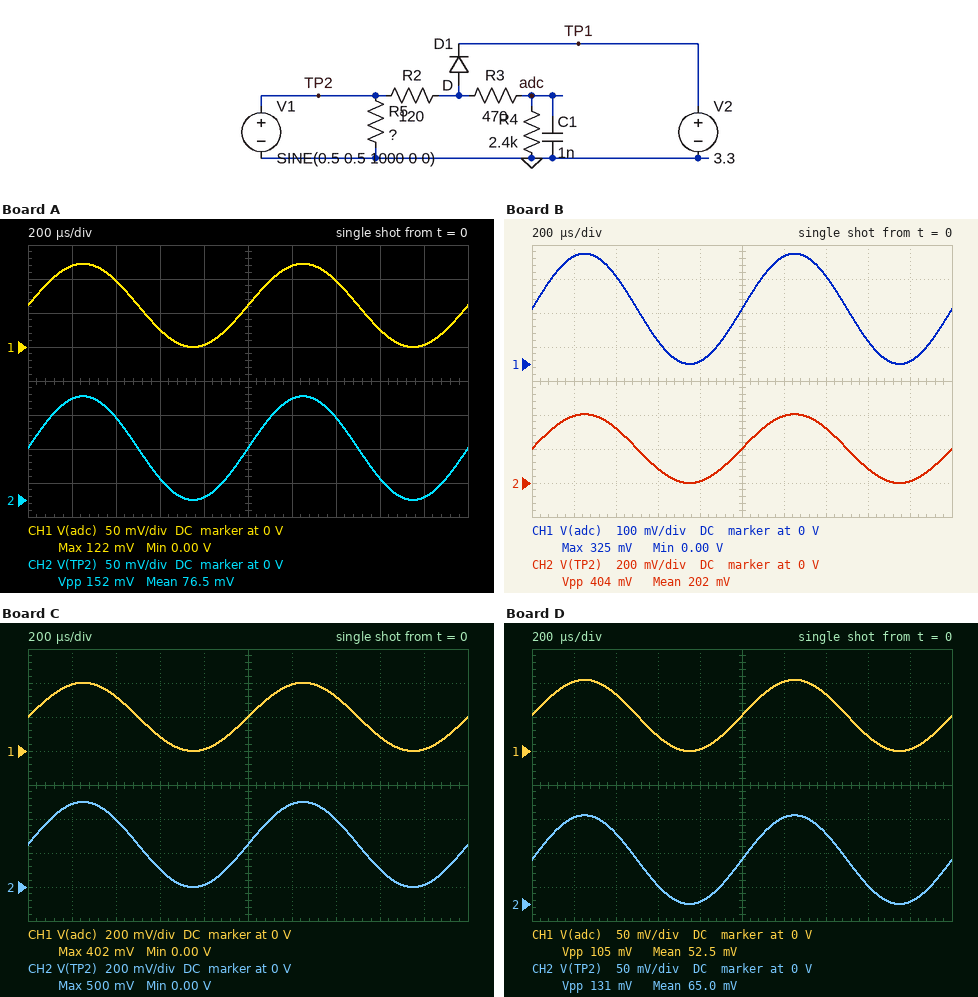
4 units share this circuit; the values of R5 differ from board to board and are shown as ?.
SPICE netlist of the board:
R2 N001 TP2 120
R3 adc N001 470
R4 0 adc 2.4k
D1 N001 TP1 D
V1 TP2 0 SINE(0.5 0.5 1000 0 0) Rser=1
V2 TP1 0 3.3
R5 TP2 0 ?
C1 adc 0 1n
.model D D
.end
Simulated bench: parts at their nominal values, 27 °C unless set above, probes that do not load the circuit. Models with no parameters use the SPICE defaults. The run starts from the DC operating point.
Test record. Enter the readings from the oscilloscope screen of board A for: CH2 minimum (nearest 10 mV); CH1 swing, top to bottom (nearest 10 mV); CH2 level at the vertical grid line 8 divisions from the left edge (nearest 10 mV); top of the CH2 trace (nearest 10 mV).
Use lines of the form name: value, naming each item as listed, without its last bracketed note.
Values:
CH2 minimum: 0 V
CH1 swing, top to bottom: 120 mV
CH2 level at the vertical grid line 8 divisions from the left edge: 30 mV
top of the CH2 trace: 150 mV
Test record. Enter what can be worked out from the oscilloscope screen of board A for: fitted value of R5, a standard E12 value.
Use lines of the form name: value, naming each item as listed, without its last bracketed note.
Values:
fitted value of R5, a standard E12 value: 0.18 Ω
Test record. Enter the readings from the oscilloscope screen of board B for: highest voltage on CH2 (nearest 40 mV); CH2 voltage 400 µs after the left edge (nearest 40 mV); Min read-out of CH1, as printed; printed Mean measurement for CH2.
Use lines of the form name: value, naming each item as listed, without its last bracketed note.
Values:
highest voltage on CH2: 400 mV
CH2 voltage 400 µs after the left edge: 320 mV
Min read-out of CH1, as printed: 0.00 V
printed Mean measurement for CH2: 202 mV
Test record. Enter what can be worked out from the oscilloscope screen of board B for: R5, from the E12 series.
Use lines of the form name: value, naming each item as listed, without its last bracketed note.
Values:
R5, from the E12 series: 0.68 Ω
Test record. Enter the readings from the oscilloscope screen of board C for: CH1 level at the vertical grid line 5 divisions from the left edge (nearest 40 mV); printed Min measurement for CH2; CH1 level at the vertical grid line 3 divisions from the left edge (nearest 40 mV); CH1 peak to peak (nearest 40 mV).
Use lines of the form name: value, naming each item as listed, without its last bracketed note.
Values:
CH1 level at the vertical grid line 5 divisions from the left edge: 200 mV
printed Min measurement for CH2: 0.00 V
CH1 level at the vertical grid line 3 divisions from the left edge: 80 mV
CH1 peak to peak: 400 mV
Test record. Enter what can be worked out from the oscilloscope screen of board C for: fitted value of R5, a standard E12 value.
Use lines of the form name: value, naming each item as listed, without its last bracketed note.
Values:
fitted value of R5, a standard E12 value: 1 Ω
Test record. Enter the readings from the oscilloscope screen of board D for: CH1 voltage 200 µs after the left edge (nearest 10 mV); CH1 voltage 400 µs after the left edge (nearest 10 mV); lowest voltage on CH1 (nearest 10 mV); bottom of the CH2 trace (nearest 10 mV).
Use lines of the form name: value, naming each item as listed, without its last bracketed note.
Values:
CH1 voltage 200 µs after the left edge: 100 mV
CH1 voltage 400 µs after the left edge: 80 mV
lowest voltage on CH1: 0 V
bottom of the CH2 trace: 0 V
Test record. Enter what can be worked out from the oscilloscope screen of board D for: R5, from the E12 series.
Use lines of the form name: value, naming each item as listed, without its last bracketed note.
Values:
R5, from the E12 series: 0.15 Ω
